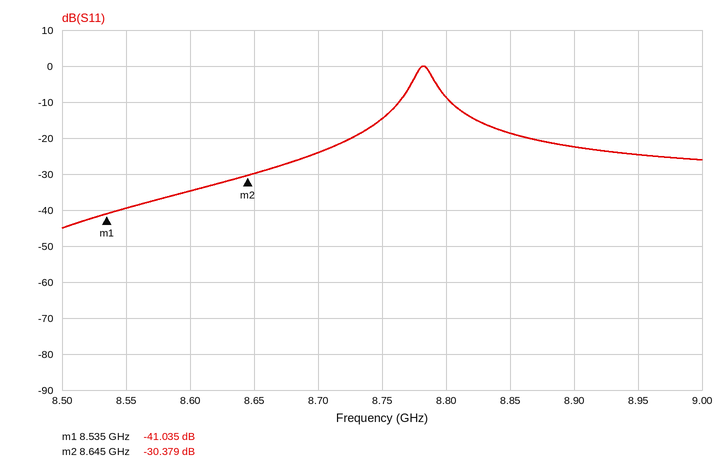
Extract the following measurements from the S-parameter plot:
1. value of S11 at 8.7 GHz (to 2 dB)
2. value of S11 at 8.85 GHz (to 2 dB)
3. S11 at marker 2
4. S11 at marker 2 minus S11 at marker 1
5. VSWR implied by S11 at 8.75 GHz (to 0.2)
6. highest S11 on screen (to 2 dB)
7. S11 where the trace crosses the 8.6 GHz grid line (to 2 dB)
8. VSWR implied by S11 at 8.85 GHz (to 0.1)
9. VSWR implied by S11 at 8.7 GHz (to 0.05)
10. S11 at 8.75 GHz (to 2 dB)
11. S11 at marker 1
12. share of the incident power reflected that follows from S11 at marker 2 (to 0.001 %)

-24 dB
-18 dB
-30.379 dB
10.656 dB
1.4
0 dB
-34 dB
1.3
1.15
-14 dB
-41.035 dB
0.092 %
